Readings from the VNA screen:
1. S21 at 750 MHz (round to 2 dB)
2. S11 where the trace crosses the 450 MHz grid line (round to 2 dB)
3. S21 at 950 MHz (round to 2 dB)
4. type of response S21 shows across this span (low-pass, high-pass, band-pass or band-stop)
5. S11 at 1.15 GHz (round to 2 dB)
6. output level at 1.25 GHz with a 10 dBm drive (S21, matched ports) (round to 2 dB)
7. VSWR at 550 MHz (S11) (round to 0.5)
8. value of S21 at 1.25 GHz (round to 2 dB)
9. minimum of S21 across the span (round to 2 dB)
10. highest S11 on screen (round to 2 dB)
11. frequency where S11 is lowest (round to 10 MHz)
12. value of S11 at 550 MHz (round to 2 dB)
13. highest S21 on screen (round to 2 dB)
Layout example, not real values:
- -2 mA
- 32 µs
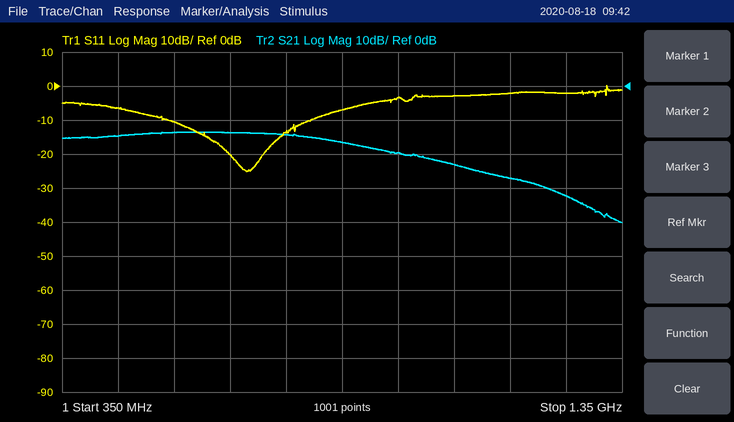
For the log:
- -14 dB
- -6 dB
- -20 dB
- low-pass
- -2 dB
- -22 dBm
- 2.0
- -32 dB
- -40 dB
- 0 dB
- 680 MHz
- -10 dB
- -14 dB
